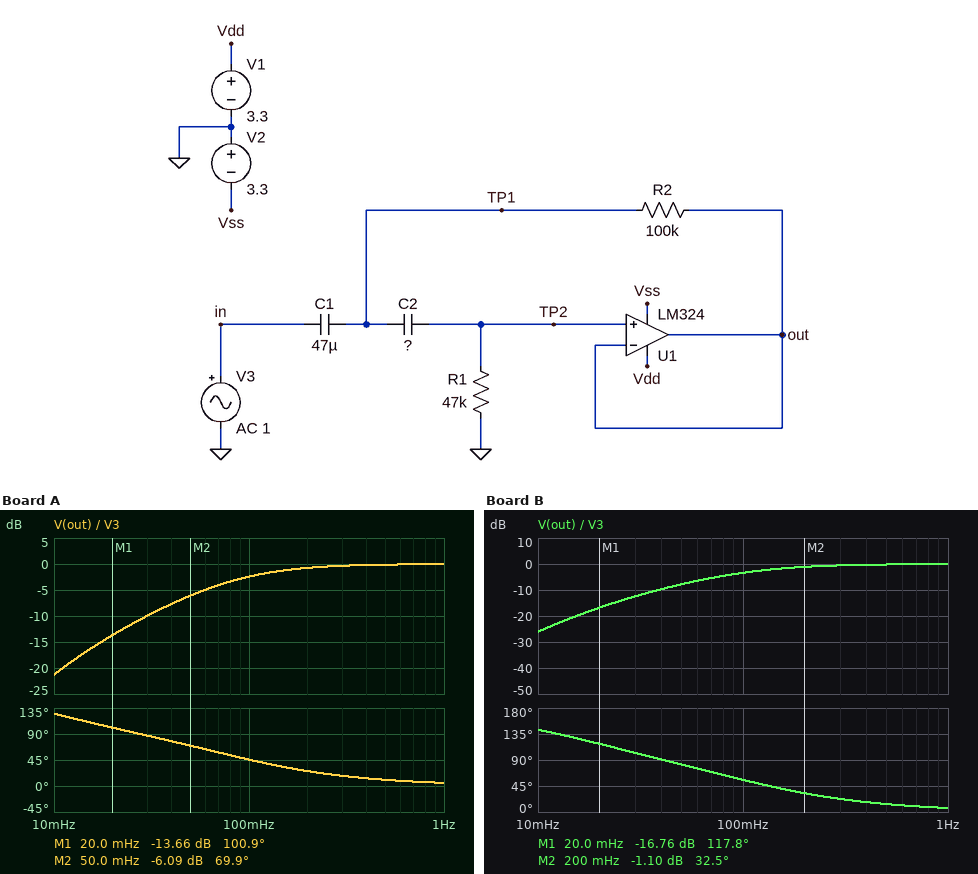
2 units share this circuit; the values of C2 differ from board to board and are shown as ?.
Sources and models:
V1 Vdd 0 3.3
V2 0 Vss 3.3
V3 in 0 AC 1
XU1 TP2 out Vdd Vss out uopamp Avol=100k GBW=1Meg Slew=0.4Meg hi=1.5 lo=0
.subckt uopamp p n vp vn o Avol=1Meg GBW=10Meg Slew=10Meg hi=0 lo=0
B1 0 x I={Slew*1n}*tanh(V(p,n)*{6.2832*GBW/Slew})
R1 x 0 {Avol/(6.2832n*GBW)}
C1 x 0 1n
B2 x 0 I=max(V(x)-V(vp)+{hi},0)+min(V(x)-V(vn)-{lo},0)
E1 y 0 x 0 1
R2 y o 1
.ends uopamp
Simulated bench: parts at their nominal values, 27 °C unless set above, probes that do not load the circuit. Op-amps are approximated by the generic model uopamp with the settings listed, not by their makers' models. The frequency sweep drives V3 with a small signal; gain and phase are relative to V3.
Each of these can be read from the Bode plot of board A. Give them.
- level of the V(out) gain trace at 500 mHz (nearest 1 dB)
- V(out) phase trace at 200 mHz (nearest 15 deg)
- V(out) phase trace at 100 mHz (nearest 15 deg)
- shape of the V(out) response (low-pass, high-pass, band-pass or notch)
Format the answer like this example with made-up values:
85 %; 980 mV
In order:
0 dB; 30 deg; 45 deg; high-pass
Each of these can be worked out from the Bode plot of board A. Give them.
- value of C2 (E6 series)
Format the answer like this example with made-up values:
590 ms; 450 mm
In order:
150 µF
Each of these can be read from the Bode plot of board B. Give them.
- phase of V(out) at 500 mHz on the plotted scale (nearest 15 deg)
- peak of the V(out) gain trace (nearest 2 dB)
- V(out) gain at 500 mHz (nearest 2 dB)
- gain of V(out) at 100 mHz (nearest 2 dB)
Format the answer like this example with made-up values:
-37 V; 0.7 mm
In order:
15 deg; 0 dB; 0 dB; -4 dB
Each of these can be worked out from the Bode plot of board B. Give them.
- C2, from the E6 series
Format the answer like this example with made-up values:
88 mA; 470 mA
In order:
68 µF
